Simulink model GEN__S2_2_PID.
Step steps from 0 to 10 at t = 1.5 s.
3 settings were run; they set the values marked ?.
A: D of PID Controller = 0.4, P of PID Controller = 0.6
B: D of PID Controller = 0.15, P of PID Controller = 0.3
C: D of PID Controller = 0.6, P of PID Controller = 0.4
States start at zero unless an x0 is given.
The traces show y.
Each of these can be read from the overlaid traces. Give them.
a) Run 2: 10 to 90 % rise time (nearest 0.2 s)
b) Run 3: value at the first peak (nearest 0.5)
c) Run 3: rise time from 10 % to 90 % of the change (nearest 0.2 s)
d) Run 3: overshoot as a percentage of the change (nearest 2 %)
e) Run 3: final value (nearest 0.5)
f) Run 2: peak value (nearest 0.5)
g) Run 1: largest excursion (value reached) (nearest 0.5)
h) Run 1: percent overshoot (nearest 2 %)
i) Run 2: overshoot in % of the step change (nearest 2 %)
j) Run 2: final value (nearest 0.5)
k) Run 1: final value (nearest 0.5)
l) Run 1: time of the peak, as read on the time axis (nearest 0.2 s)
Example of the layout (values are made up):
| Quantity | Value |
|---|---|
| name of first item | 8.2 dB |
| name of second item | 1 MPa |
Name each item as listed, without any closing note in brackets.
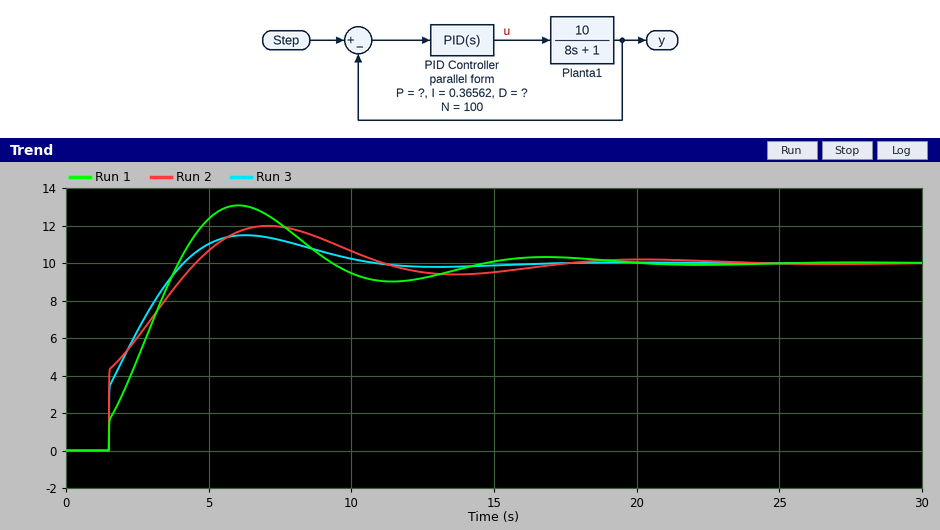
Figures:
| Quantity | Value |
|---|---|
| Run 2: 10 to 90 % rise time | 2.4 s |
| Run 3: value at the first peak | 11.5 |
| Run 3: rise time from 10 % to 90 % of the change | 2.0 s |
| Run 3: overshoot as a percentage of the change | 14 % |
| Run 3: final value | 10.0 |
| Run 2: peak value | 12.0 |
| Run 1: largest excursion (value reached) | 13.0 |
| Run 1: percent overshoot | 30 % |
| Run 2: overshoot in % of the step change | 20 % |
| Run 2: final value | 10.0 |
| Run 1: final value | 10.0 |
| Run 1: time of the peak, as read on the time axis | 6.0 s |
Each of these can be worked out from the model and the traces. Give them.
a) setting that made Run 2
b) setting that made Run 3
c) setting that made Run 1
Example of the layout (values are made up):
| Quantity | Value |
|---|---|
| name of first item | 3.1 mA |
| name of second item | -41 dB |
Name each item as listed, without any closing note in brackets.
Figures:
| Quantity | Value |
|---|---|
| setting that made Run 2 | C |
| setting that made Run 3 | A |
| setting that made Run 1 | B |
